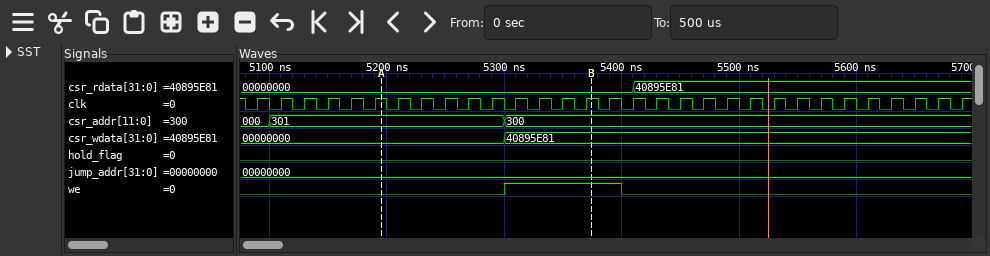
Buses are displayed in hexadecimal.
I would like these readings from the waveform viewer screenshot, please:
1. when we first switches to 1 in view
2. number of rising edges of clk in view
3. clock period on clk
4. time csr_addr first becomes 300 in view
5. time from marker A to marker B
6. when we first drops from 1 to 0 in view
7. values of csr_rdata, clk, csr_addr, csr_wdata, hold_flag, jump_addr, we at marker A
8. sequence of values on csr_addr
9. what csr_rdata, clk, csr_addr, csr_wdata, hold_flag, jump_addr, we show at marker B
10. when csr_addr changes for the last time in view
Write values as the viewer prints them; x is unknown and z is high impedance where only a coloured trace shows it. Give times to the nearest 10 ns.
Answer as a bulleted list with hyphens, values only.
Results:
- 5300 ns
- 31
- 20 ns
- 5300 ns
- 180 ns
- 5400 ns
- csr_rdata=00000000, clk=1, csr_addr=301, csr_wdata=00000000, hold_flag=0, jump_addr=00000000, we=0
- 000, 301, 300
- csr_rdata=00000000, clk=1, csr_addr=300, csr_wdata=40895E81, hold_flag=0, jump_addr=00000000, we=1
- 5300 ns
